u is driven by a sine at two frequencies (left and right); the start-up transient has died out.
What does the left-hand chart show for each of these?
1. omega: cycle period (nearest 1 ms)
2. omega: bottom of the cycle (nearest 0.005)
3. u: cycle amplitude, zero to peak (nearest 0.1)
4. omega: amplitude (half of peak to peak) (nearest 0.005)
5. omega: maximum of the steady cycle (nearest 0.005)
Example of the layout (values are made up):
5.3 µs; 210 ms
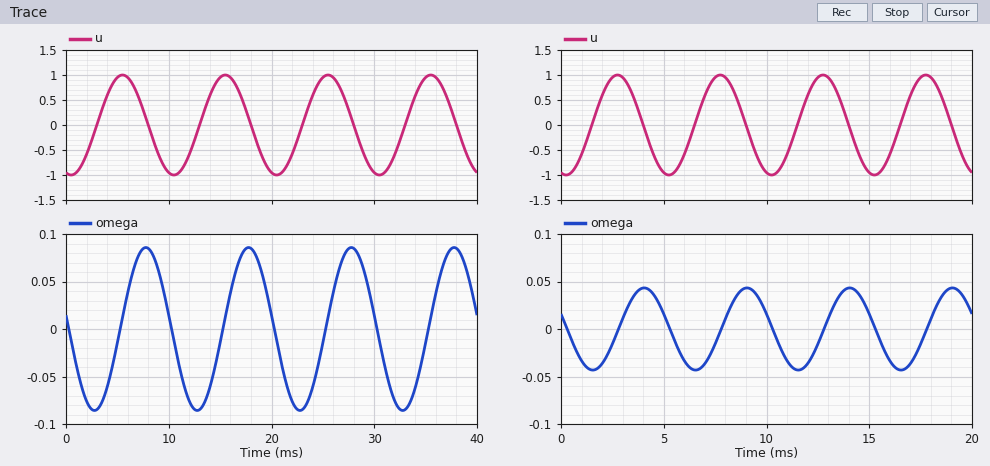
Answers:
10 ms; -0.085; 1.0; 0.085; 0.085
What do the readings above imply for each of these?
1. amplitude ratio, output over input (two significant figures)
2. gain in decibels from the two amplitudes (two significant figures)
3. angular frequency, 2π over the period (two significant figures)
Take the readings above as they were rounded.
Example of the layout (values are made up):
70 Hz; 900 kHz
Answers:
0.085; -21 dB; 0.63 rad/ms
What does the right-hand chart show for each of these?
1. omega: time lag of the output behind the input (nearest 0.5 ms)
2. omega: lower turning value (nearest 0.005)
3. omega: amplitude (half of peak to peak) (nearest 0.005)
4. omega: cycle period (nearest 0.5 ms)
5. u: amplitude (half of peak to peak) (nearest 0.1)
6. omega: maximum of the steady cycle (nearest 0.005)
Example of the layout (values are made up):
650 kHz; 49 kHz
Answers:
1.5 ms; -0.045; 0.045; 5.0 ms; 1.0; 0.045
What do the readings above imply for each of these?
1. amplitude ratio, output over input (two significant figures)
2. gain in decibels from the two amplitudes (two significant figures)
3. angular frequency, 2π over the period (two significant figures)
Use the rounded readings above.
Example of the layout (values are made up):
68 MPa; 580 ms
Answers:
0.045; -27 dB; 1.3 rad/ms
